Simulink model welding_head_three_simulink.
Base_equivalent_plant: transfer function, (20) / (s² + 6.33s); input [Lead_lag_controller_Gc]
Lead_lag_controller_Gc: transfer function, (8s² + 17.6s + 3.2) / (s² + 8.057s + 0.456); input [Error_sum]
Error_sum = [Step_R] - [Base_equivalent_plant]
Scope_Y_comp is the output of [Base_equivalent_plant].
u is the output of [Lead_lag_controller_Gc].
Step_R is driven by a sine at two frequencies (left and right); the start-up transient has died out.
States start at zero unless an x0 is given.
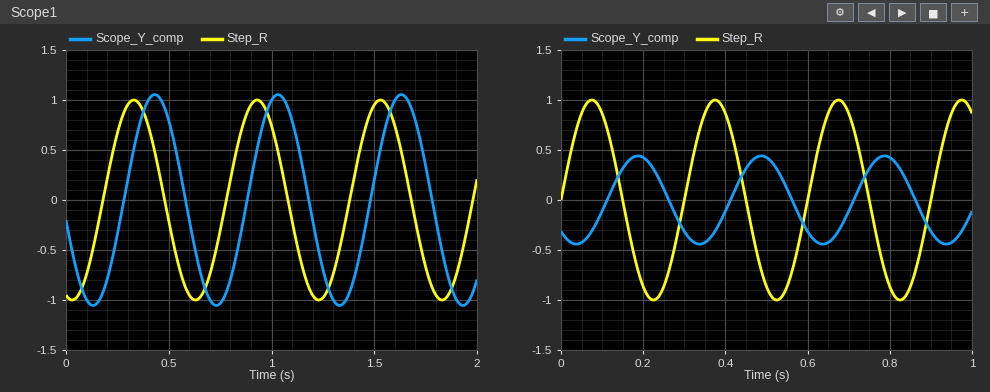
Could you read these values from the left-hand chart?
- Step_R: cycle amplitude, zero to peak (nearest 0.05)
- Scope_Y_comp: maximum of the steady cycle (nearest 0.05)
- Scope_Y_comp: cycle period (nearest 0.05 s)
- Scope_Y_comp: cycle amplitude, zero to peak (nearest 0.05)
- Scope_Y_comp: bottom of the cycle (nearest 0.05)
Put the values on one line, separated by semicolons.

1.00; 1.05; 0.60 s; 1.05; -1.05
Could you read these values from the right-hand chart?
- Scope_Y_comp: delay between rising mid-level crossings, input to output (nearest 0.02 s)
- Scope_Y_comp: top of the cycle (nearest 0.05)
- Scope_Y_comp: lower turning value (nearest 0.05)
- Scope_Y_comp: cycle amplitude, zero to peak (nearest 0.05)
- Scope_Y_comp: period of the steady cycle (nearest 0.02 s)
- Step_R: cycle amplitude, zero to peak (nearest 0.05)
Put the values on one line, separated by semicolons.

0.12 s; 0.45; -0.45; 0.45; 0.30 s; 1.00
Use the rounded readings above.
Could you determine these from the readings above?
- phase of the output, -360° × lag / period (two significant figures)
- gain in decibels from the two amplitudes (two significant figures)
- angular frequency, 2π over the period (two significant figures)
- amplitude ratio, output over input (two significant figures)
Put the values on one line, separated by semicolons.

-140°; -6.9 dB; 21 rad/s; 0.45
